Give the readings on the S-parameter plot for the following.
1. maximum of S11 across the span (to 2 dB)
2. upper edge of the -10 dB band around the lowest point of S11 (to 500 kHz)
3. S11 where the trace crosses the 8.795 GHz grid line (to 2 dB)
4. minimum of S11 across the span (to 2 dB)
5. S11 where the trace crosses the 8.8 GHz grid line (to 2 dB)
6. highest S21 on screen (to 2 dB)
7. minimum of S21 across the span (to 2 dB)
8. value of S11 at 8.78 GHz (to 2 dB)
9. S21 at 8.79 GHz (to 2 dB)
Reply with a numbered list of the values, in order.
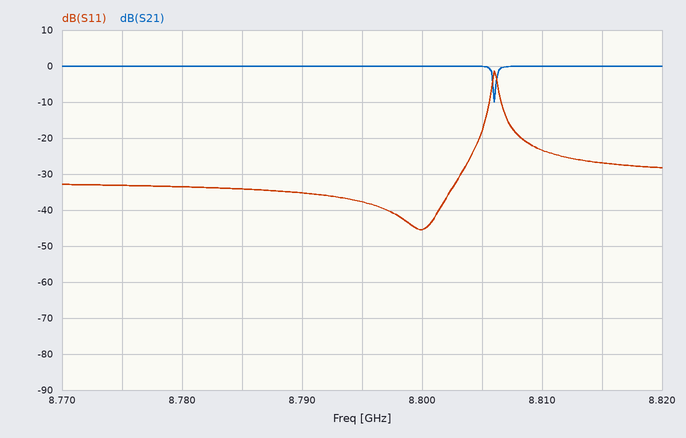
1. -2 dB
2. 8.8055 GHz
3. -38 dB
4. -46 dB
5. -46 dB
6. 0 dB
7. -10 dB
8. -34 dB
9. 0 dB
